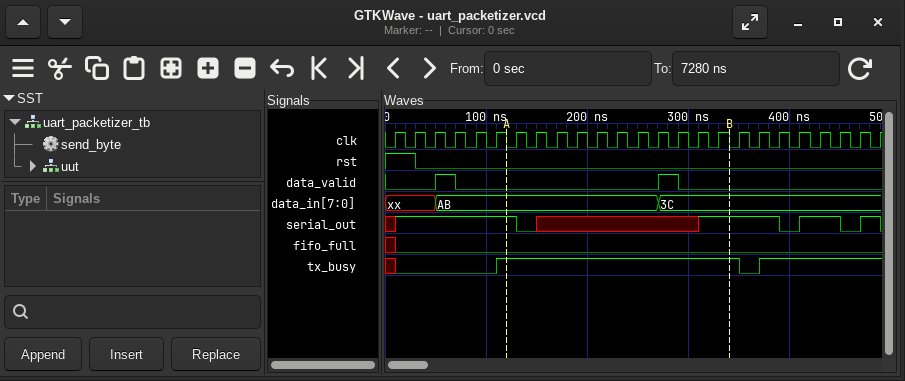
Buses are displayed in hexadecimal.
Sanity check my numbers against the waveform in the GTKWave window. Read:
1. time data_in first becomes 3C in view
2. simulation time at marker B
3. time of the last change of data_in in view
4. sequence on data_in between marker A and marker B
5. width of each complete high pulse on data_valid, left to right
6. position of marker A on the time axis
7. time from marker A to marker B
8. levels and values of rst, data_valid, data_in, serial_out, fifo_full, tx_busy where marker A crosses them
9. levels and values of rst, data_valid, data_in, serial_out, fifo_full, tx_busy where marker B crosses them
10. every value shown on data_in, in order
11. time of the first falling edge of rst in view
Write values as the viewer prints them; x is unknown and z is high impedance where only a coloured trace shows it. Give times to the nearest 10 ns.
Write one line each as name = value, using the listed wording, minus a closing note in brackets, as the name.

time data_in first becomes 3C in view = 270 ns
simulation time at marker B = 340 ns
time of the last change of data_in in view = 270 ns
sequence on data_in between marker A and marker B = AB, 3C
width of each complete high pulse on data_valid, left to right = 20 ns, 20 ns
position of marker A on the time axis = 120 ns
time from marker A to marker B = 220 ns
levels and values of rst, data_valid, data_in, serial_out, fifo_full, tx_busy where marker A crosses them = rst=0, data_valid=0, data_in=AB, serial_out=1, fifo_full=0, tx_busy=1
levels and values of rst, data_valid, data_in, serial_out, fifo_full, tx_busy where marker B crosses them = rst=0, data_valid=0, data_in=3C, serial_out=1, fifo_full=0, tx_busy=1
every value shown on data_in, in order = xx, AB, 3C
time of the first falling edge of rst in view = 30 ns
